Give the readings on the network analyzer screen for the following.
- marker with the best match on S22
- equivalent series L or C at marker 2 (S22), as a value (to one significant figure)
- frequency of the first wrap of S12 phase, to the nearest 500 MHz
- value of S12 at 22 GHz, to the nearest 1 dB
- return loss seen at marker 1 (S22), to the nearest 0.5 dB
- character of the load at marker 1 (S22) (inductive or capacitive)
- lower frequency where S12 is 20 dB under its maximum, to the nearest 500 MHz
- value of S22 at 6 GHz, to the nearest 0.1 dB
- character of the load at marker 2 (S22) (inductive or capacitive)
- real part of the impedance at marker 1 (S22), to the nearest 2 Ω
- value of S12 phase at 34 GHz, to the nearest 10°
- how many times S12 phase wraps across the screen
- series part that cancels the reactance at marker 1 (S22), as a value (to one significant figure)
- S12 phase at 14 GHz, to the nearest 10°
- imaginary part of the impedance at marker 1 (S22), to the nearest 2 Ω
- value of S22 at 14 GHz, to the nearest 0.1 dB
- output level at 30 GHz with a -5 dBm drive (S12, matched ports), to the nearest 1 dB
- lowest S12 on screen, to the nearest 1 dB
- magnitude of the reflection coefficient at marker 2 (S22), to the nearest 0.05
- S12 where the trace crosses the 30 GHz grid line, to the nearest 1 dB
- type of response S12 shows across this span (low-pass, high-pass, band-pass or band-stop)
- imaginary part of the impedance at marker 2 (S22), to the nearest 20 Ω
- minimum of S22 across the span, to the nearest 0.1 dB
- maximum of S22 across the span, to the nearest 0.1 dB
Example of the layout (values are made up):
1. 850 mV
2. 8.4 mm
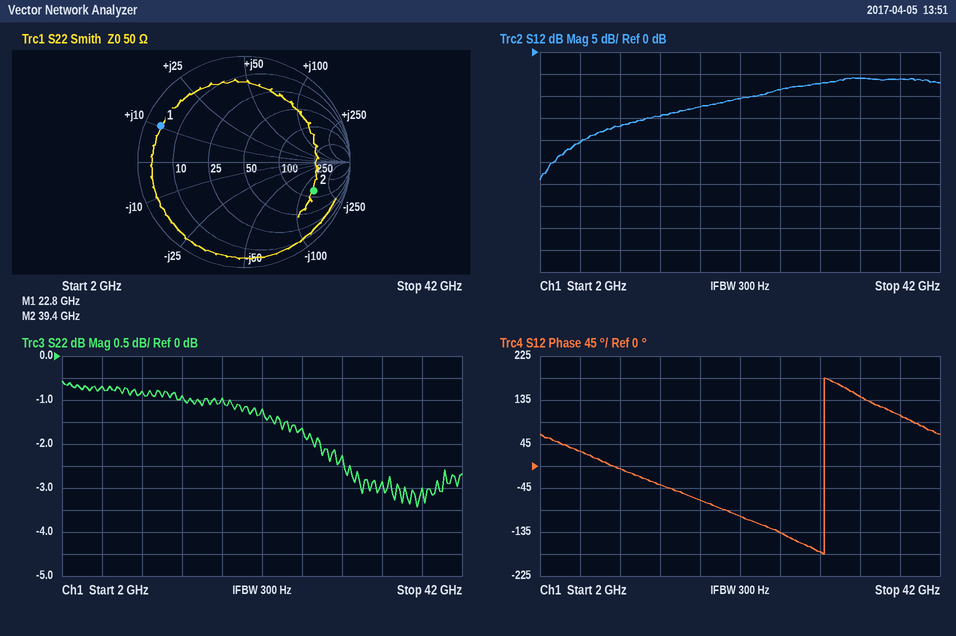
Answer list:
1. marker 2
2. 30 fF
3. 30.5 GHz
4. -11 dB
5. 1.5 dB
6. inductive
7. 3.0 GHz
8. -0.7 dB
9. capacitive
10. 4 Ω
11. 140°
12. 1
13. 700 fF
14. -40°
15. +10 Ω
16. -0.9 dB
17. -12 dBm
18. -29 dB
19. 0.70
20. -7 dB
21. high-pass
22. -140 Ω
23. -3.4 dB
24. -0.6 dB
